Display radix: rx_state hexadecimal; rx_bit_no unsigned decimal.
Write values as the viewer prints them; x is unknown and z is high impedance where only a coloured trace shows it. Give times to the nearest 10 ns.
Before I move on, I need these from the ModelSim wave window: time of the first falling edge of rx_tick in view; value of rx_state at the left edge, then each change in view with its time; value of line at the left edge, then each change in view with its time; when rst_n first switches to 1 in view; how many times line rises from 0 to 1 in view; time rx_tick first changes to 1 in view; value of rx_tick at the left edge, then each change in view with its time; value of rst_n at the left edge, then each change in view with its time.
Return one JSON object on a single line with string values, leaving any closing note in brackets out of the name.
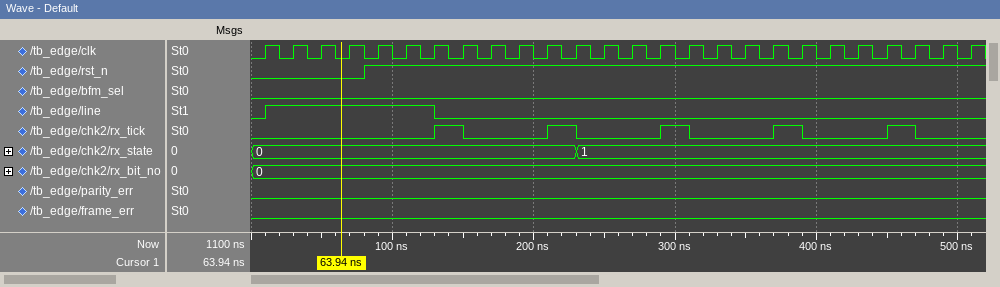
{"time of the first falling edge of rx_tick in view": "150 ns", "value of rx_state at the left edge, then each change in view with its time": "0, 1 at 230 ns", "value of line at the left edge, then each change in view with its time": "0, 1 at 10 ns, 0 at 130 ns", "when rst_n first switches to 1 in view": "80 ns", "how many times line rises from 0 to 1 in view": "1", "time rx_tick first changes to 1 in view": "130 ns", "value of rx_tick at the left edge, then each change in view with its time": "0, 1 at 130 ns, 0 at 150 ns, 1 at 210 ns, 0 at 230 ns, 1 at 290 ns, 0 at 310 ns, 1 at 370 ns, 0 at 390 ns, 1 at 450 ns, 0 at 470 ns", "value of rst_n at the left edge, then each change in view with its time": "0, 1 at 80 ns"}
